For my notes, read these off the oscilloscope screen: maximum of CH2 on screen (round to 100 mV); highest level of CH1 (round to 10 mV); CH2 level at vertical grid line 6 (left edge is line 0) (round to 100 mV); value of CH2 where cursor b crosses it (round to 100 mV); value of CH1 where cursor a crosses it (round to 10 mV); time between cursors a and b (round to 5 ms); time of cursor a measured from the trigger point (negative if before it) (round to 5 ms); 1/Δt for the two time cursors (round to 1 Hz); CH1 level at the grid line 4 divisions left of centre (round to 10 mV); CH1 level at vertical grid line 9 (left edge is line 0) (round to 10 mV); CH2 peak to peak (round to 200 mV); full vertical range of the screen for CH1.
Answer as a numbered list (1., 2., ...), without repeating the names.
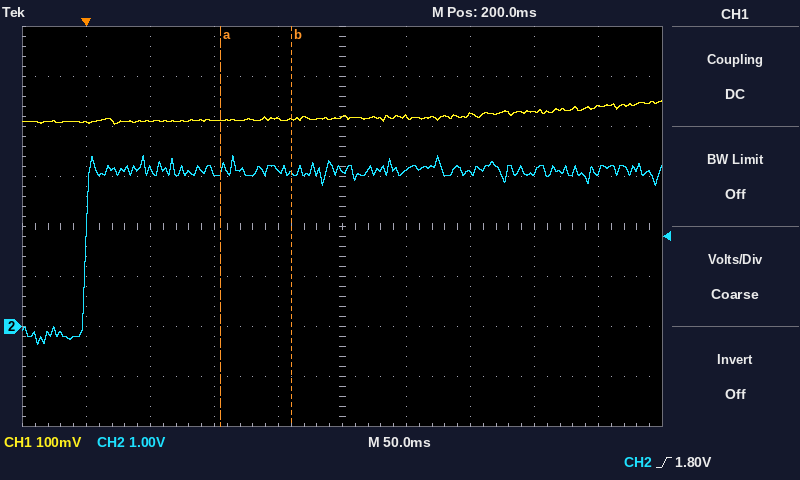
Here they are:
1. 3.4 V
2. 450 mV
3. 3.1 V
4. 3.1 V
5. 410 mV
6. 55 ms
7. +105 ms
8. 18 Hz
9. 410 mV
10. 440 mV
11. 3.8 V
12. 800 mV
